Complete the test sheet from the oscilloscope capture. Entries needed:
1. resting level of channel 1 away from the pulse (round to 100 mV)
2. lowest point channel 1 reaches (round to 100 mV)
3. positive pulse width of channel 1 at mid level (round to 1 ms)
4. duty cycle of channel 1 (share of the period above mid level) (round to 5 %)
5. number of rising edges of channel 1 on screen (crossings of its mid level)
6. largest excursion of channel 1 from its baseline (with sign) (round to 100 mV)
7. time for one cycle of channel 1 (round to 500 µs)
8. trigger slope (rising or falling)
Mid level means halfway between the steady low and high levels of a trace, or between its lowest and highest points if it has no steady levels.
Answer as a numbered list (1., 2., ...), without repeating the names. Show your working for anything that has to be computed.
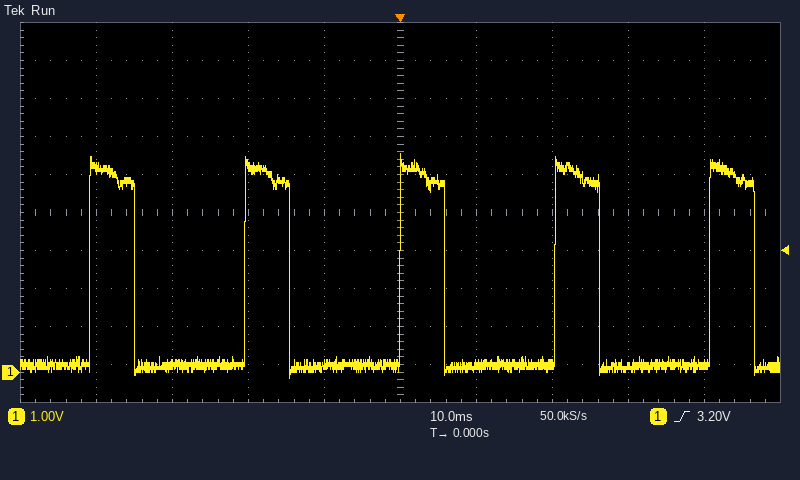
1. 200 mV
2. -200 mV
3. 6 ms
4. 6 ms / 20.5 ms ≈ 29.3 %, so 30 % to the nearest 5 %
5. 5
6. +5.6 V
7. 20.5 ms
8. rising
